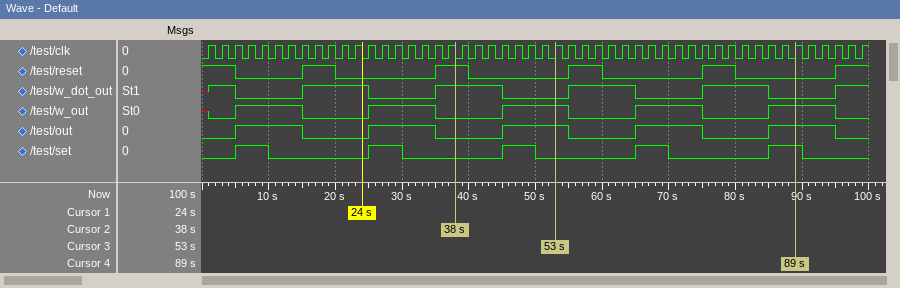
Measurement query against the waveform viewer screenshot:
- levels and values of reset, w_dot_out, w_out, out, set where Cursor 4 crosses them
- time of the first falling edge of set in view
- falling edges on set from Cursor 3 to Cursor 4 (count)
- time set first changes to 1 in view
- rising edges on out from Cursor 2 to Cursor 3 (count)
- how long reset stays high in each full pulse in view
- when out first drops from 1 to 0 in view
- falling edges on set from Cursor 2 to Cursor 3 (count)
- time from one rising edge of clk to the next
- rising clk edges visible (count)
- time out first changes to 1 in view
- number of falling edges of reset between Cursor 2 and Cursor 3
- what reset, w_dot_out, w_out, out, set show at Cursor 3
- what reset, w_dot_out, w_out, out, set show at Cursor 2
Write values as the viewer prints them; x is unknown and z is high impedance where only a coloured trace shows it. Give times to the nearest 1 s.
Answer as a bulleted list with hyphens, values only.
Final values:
- reset=0, w_dot_out=0, w_out=1, out=1, set=1
- 10 s
- 1
- 5 s
- 1
- 5 s, 5 s, 5 s, 5 s
- 15 s
- 1
- 2 s
- 50
- 5 s
- 1
- reset=0, w_dot_out=0, w_out=1, out=1, set=0
- reset=1, w_dot_out=1, w_out=0, out=0, set=0
